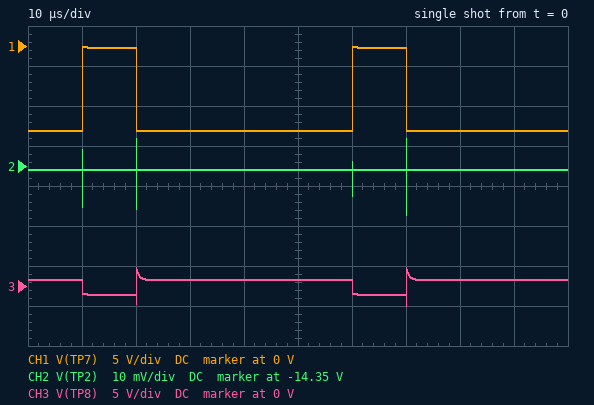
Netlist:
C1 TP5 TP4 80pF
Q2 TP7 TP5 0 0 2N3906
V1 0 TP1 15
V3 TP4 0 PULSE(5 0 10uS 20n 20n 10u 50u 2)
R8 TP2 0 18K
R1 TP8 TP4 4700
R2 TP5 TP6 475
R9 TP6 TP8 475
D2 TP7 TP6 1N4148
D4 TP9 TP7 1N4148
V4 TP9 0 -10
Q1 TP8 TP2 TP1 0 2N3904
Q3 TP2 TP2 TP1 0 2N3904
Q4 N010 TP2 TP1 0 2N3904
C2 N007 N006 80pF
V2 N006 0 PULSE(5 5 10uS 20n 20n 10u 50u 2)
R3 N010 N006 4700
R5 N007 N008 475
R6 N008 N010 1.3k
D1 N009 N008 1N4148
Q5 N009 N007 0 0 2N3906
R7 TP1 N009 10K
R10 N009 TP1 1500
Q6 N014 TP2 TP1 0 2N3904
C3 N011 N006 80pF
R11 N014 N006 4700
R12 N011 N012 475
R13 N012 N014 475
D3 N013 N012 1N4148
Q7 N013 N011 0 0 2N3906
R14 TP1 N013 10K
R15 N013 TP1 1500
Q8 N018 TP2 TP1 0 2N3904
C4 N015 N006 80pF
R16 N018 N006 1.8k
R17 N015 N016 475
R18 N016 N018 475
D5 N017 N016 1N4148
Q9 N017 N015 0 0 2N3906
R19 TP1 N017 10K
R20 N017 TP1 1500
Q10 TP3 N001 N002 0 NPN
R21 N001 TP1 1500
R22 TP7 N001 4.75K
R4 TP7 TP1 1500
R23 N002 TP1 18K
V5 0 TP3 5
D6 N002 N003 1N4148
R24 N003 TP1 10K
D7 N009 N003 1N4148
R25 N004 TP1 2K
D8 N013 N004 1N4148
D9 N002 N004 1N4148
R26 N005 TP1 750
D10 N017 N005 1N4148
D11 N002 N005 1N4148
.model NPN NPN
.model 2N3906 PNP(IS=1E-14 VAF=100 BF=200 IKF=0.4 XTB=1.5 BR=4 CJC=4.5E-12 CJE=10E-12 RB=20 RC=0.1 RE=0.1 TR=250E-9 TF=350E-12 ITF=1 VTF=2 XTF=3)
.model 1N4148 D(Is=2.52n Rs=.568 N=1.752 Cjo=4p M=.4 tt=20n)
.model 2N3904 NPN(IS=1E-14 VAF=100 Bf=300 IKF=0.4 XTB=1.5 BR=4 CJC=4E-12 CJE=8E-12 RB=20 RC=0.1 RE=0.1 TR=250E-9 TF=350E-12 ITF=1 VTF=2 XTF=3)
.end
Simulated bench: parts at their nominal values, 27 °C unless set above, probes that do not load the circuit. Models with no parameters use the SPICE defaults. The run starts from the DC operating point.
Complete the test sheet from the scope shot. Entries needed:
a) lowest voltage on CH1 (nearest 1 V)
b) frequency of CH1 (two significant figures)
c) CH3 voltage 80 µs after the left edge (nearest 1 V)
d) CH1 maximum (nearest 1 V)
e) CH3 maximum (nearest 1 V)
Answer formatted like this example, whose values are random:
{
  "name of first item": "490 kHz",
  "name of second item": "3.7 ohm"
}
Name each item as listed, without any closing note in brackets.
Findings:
{
  "lowest voltage on CH1": "-11 V",
  "frequency of CH1": "20 kHz",
  "CH3 voltage 80 µs after the left edge": "1 V",
  "CH1 maximum": "0 V",
  "CH3 maximum": "2 V"
}
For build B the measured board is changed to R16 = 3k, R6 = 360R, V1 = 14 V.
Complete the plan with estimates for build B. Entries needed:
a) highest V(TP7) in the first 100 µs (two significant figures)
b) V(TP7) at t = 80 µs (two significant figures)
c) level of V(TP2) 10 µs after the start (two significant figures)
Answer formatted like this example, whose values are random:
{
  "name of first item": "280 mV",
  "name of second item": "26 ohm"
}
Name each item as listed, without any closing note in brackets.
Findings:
{
  "highest V(TP7) in the first 100 µs": "-80 mV",
  "V(TP7) at t = 80 µs": "-11 V",
  "level of V(TP2) 10 µs after the start": "-13 V"
}
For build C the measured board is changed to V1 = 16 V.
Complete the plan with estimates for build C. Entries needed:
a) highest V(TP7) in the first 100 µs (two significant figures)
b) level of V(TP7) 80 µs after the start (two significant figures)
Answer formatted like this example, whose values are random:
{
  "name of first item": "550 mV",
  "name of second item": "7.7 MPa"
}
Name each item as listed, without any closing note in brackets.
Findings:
{
  "highest V(TP7) in the first 100 µs": "-77 mV",
  "level of V(TP7) 80 µs after the start": "-11 V"
}
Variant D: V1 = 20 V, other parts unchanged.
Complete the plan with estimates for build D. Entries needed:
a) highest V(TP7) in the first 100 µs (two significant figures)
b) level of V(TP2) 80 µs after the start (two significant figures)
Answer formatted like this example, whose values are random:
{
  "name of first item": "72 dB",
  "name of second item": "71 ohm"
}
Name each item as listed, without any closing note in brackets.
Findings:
{
  "highest V(TP7) in the first 100 µs": "-74 mV",
  "level of V(TP2) 80 µs after the start": "-19 V"
}
